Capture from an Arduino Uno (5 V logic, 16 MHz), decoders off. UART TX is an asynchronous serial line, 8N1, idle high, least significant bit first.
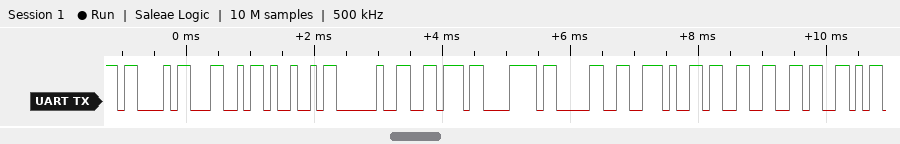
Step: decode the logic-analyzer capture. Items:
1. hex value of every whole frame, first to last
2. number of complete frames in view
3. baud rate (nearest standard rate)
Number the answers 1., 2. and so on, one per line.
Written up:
1. 0x43 0x4C 0x49 0x20 0x76 0x78 0x30 0x2E 0x33 0x36
2. 10
3. 9600 baud
